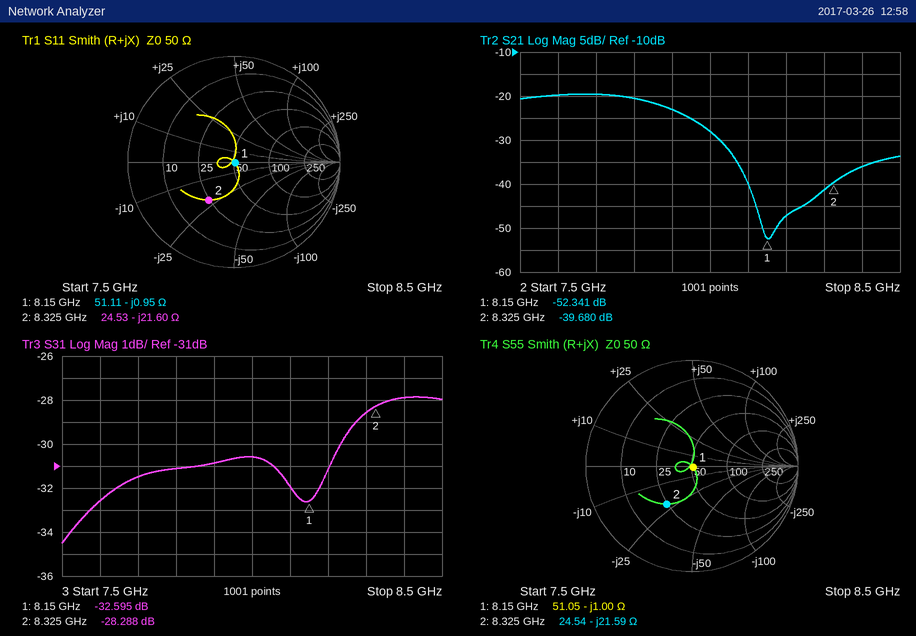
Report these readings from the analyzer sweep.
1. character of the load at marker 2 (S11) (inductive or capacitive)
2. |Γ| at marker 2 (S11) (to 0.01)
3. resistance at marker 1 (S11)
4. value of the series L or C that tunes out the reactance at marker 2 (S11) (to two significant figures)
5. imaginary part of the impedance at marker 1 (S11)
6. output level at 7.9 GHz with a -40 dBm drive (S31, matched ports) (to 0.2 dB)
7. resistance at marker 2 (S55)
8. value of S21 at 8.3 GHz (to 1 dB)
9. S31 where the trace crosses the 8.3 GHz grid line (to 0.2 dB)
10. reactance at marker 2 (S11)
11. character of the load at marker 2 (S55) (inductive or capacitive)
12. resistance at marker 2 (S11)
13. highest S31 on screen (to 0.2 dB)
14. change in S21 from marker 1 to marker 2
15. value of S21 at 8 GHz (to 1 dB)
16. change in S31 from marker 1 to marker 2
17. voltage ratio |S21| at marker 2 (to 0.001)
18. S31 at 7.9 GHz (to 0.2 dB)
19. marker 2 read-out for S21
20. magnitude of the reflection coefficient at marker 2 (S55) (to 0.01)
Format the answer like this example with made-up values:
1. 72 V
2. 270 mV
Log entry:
1. capacitive
2. 0.43
3. 51.11 Ω
4. 410 pH
5. -0.95 Ω
6. -70.8 dBm
7. 24.54 Ω
8. -41 dB
9. -28.6 dB
10. -21.60 Ω
11. capacitive
12. 24.53 Ω
13. -27.8 dB
14. 12.661 dB
15. -28 dB
16. 4.307 dB
17. 0.010
18. -30.8 dB
19. -39.680 dB
20. 0.43
